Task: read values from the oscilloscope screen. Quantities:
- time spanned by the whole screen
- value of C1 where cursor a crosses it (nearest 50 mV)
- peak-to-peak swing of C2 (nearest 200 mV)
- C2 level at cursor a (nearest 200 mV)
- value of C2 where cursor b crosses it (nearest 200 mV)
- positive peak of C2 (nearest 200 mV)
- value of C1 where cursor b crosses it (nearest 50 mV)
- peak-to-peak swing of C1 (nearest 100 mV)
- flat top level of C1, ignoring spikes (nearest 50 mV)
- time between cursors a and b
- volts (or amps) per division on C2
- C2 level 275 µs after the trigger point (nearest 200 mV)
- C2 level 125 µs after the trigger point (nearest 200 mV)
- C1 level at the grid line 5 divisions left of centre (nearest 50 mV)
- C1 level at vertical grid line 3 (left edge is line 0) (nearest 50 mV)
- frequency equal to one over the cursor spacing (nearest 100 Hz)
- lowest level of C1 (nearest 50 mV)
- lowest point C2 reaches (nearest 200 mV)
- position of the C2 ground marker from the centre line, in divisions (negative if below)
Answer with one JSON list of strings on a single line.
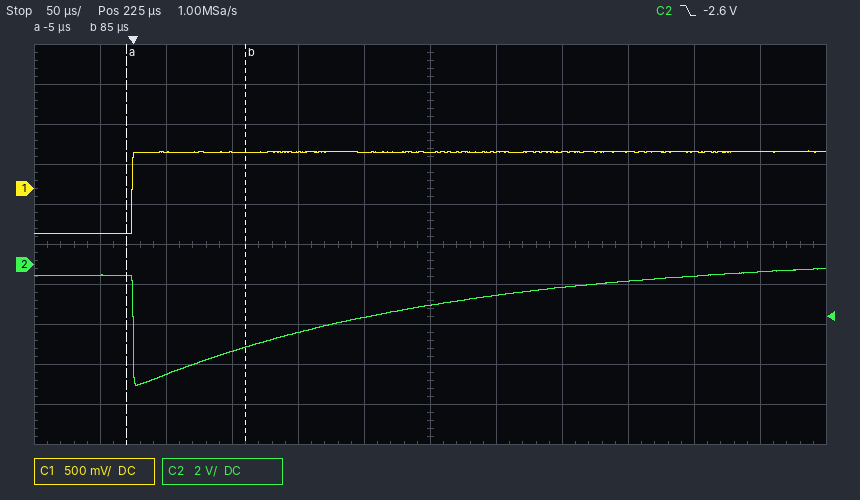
["600 µs", "-550 mV", "5.8 V", "-600 mV", "-4.2 V", "-200 mV", "450 mV", "1.00 V", "450 mV", "90 µs", "2 V", "-1.6 V", "-3.4 V", "-550 mV", "450 mV", "11.1 kHz", "-550 mV", "-6.0 V", "-0.5 div"]
